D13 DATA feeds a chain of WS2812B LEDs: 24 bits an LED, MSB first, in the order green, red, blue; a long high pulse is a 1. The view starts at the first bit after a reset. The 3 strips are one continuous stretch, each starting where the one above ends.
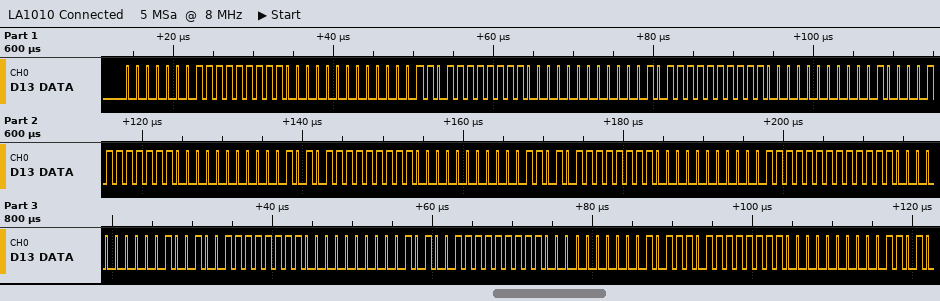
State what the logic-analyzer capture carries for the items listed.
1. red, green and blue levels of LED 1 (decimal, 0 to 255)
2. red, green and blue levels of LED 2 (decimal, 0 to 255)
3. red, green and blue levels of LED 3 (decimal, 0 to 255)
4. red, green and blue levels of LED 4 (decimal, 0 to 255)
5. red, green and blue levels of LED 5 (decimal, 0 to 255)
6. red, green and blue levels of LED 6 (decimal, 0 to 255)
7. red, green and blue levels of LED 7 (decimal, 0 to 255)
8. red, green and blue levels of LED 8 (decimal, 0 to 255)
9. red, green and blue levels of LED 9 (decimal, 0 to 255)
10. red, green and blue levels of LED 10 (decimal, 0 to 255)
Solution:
255, 1, 0
255, 6, 0
255, 11, 0
255, 16, 0
255, 21, 0
255, 26, 0
255, 31, 0
255, 36, 0
255, 41, 0
255, 46, 0
